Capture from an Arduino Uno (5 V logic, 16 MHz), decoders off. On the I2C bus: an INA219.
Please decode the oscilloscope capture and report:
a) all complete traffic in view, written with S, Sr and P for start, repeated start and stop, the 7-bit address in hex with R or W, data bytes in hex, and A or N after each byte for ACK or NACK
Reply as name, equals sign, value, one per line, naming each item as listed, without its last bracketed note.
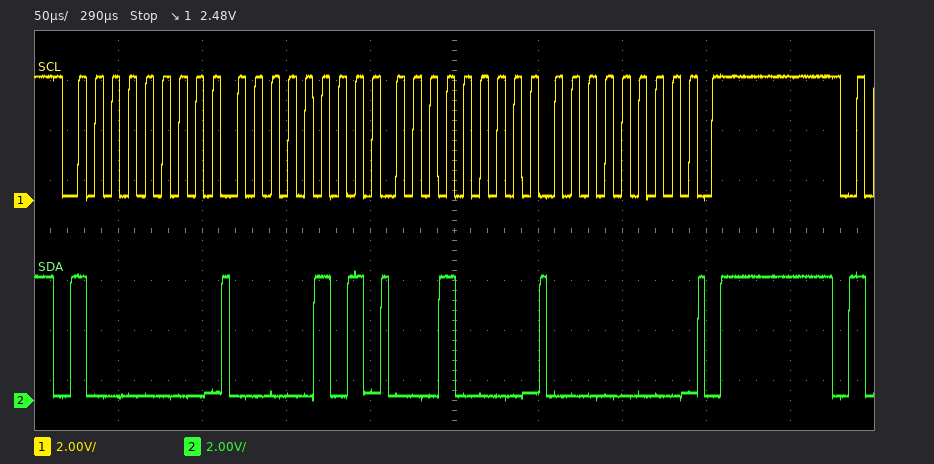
all complete traffic in view, written with S, Sr and P for start, repeated start and stop, the 7-bit address in hex with R or W, data bytes in hex, and A or N after each byte for ACK or NACK = S 40W A 05 A 10 A 00 A P
